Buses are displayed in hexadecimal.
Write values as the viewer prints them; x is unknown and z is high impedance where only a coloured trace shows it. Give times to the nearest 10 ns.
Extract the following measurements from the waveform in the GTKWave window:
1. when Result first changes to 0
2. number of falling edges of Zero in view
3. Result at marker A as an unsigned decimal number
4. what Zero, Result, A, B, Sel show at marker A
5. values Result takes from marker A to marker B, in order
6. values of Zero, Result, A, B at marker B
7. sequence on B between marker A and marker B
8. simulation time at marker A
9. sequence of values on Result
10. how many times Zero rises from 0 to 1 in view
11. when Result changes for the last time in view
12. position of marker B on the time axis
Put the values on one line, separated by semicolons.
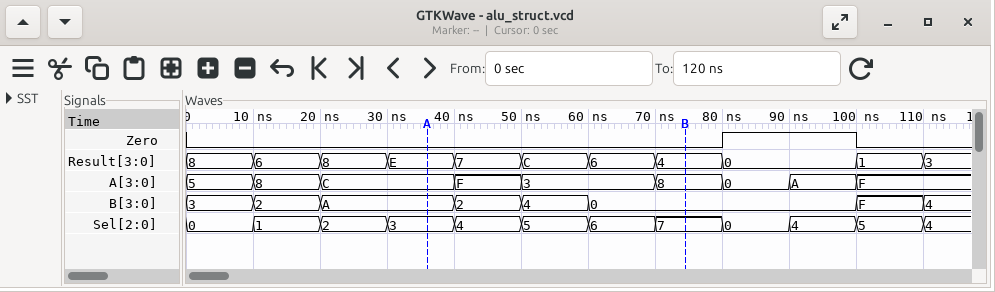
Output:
80 ns; 1; 14; Zero=0, Result=E, A=C, B=A, Sel=3; E, 7, C, 6, 4; Zero=0, Result=4, A=8, B=0; A, 2, 4, 0; 40 ns; 8, 6, 8, E, 7, C, 6, 4, 0, 1, 3; 1; 110 ns; 70 ns
